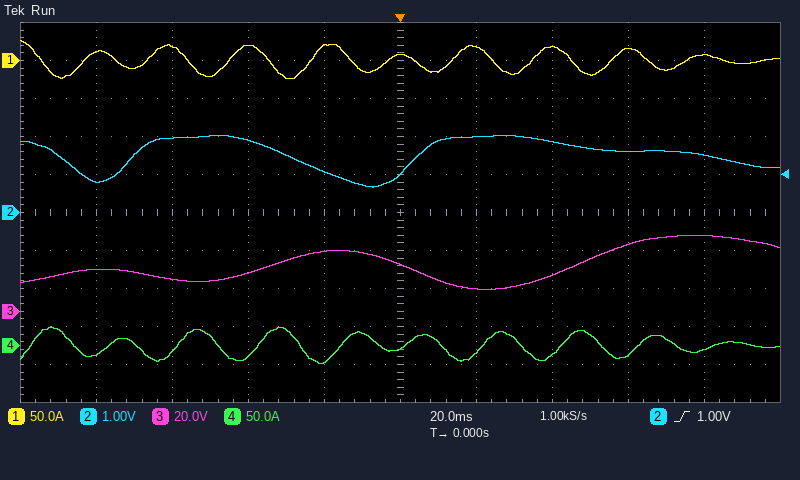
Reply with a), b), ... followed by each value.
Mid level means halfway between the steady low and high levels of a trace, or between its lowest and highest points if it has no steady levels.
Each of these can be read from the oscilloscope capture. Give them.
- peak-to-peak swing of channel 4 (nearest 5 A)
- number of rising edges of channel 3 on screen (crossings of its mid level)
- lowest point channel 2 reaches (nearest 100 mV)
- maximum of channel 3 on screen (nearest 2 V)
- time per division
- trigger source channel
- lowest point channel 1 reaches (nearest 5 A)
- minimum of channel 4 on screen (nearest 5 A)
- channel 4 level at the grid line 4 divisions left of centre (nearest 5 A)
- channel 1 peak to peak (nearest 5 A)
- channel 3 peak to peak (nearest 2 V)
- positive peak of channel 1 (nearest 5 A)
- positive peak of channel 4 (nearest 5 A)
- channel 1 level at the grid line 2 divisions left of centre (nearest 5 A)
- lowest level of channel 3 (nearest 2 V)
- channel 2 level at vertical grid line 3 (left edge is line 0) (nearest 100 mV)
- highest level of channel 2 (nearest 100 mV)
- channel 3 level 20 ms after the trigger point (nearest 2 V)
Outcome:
a) 50 A
b) 2
c) 700 mV
d) 40 V
e) 20 ms
f) channel 2
g) -25 A
h) -25 A
i) -10 A
j) 50 A
k) 28 V
l) 25 A
m) 25 A
n) 20 A
o) 12 V
p) 1.9 V
q) 2.0 V
r) 12 V
